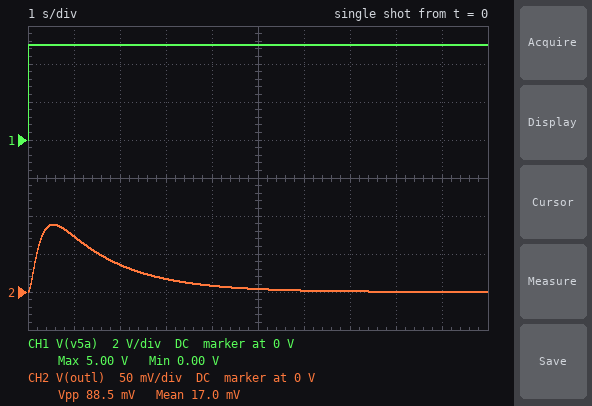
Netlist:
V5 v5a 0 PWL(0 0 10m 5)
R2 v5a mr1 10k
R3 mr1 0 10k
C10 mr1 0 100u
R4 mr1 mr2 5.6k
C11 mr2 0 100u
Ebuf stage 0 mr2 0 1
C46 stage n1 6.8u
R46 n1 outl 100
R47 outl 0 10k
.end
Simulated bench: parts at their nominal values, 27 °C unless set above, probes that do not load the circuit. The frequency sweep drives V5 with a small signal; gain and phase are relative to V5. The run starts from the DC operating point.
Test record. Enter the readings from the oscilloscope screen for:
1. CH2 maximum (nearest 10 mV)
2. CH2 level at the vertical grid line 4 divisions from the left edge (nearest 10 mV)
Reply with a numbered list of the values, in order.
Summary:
1. 90 mV
2. 10 mV
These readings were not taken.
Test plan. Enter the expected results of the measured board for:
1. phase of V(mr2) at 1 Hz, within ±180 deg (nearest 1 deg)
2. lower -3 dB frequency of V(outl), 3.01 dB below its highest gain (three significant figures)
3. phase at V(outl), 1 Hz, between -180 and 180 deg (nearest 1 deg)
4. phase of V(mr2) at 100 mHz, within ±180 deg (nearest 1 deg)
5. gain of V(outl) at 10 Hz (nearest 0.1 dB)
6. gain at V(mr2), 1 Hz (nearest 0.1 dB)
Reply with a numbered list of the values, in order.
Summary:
1. -136 deg
2. 91.3 mHz
3. -69 deg
4. -48 deg
5. -67.2 dB
6. -29.0 dB
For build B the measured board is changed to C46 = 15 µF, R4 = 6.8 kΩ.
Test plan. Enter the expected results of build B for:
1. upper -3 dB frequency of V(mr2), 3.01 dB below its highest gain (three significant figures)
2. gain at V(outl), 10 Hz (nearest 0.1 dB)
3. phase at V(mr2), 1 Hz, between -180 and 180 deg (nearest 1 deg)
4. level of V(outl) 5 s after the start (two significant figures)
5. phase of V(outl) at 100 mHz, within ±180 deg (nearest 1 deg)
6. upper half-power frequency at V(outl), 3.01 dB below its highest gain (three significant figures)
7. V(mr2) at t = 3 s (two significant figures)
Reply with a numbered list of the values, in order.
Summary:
1. 107 mHz
2. -68.7 dB
3. -140 deg
4. 11 mV
5. 34 deg
6. 671 mHz
7. 2.1 V
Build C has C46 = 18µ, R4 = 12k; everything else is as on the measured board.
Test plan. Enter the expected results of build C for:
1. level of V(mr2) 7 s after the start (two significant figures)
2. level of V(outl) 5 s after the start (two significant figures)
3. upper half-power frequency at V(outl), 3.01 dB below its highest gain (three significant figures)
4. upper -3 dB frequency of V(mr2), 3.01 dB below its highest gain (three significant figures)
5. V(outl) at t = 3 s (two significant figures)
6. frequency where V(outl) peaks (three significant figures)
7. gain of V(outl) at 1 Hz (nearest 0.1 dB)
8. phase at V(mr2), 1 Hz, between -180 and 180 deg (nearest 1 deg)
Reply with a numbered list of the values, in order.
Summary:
1. 2.4 V
2. 22 mV
3. 517 mHz
4. 82.3 mHz
5. 65 mV
6. 188 mHz
7. -37.1 dB
8. -149 deg
